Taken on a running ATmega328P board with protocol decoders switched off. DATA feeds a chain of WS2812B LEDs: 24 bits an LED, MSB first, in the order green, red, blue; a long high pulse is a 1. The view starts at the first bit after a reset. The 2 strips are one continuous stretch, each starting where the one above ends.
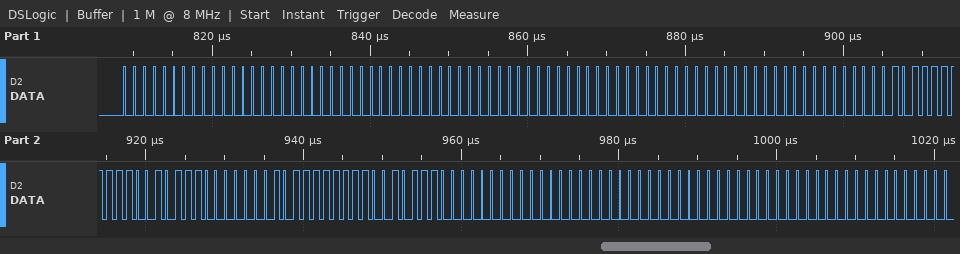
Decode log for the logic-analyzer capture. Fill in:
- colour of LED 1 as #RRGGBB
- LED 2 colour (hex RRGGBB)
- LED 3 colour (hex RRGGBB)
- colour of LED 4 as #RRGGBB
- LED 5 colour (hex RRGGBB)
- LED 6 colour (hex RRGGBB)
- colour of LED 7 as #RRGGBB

#000000
#000000
#000000
#FF022E
#FF022E
#000000
#000000
